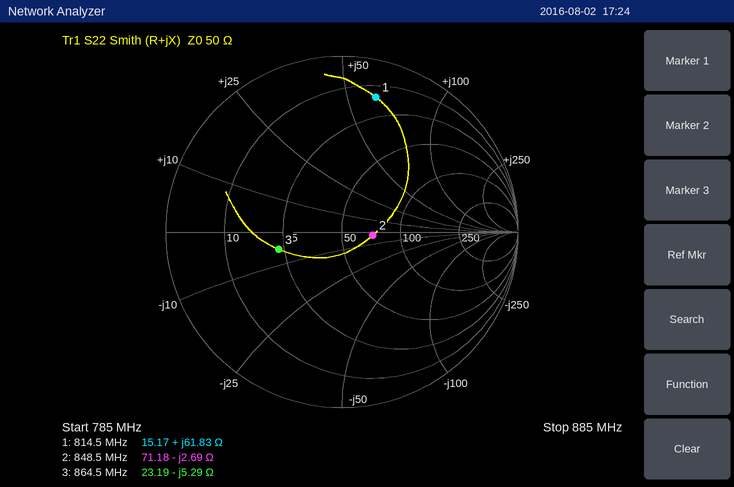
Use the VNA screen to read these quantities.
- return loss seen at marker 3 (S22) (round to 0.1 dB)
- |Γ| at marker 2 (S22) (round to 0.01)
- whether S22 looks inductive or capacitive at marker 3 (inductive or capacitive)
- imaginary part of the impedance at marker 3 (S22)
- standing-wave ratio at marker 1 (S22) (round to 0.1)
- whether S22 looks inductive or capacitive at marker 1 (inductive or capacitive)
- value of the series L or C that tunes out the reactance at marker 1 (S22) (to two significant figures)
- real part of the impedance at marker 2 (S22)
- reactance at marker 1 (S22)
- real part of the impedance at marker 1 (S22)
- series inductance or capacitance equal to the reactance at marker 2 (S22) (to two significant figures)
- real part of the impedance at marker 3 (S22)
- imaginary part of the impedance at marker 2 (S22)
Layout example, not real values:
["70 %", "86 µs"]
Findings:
["8.6 dB", "0.18", "capacitive", "-5.29 Ω", "8.5", "inductive", "3.2 pF", "71.18 Ω", "+61.83 Ω", "15.17 Ω", "70 pF", "23.19 Ω", "-2.69 Ω"]
